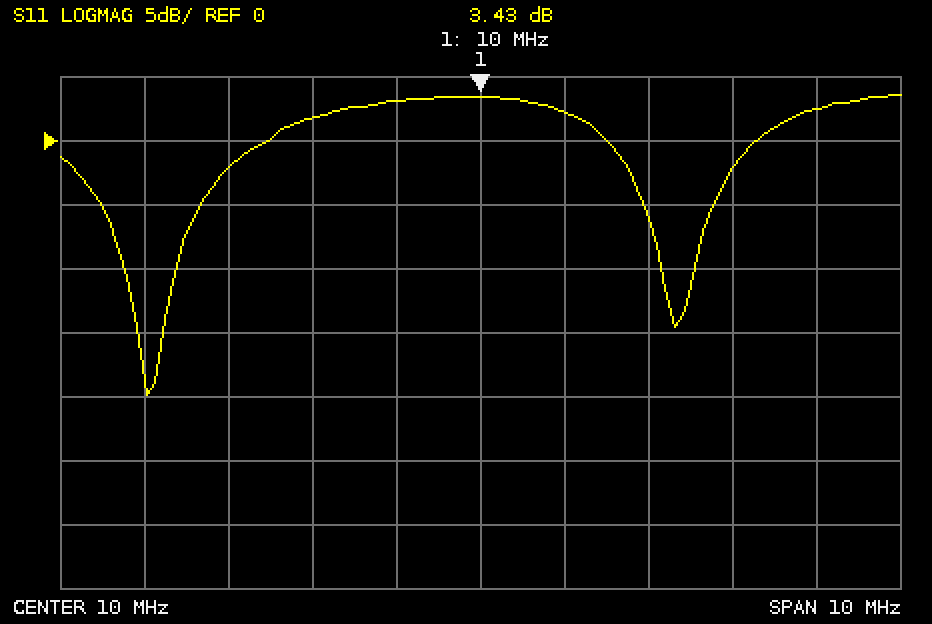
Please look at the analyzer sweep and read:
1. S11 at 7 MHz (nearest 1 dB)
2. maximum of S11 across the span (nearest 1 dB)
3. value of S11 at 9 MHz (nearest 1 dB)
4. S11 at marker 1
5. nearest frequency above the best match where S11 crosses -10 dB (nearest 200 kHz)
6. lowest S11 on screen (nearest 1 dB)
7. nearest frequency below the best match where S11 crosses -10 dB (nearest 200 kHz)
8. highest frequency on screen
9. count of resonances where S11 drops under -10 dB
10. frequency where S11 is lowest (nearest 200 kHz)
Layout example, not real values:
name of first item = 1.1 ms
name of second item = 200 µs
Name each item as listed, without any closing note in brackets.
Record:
S11 at 7 MHz = -2 dB
maximum of S11 across the span = 4 dB
value of S11 at 9 MHz = 3 dB
S11 at marker 1 = 3.43 dB
nearest frequency above the best match where S11 crosses -10 dB = 6.4 MHz
lowest S11 on screen = -20 dB
nearest frequency below the best match where S11 crosses -10 dB = 5.8 MHz
highest frequency on screen = 15 MHz
count of resonances where S11 drops under -10 dB = 2
frequency where S11 is lowest = 6.0 MHz
